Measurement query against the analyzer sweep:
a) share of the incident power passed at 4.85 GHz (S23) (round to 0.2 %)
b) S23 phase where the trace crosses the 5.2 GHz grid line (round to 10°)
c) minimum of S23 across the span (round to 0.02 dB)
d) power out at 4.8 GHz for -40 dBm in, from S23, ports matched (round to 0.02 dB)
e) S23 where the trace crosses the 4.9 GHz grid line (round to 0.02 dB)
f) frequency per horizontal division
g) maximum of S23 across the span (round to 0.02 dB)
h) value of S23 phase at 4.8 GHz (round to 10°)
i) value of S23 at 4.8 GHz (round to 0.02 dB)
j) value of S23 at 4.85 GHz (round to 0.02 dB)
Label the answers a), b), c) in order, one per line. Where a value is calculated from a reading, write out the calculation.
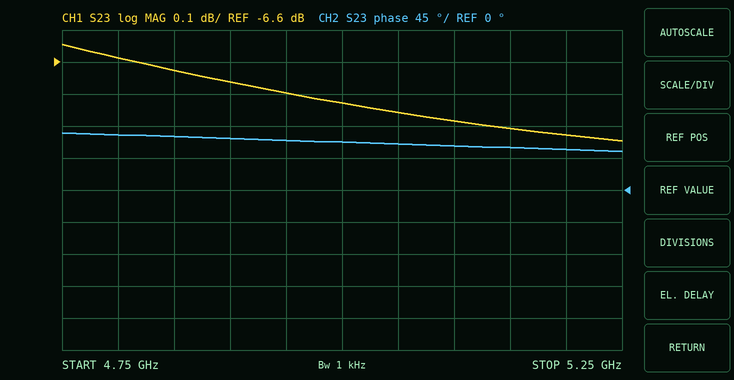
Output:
a) 10^(-6.62/10) ≈ 21.8 %
b) 60°
c) -6.84 dB
d) -40 dBm + (-6.58 dB) = -46.58 dBm
e) -6.66 dB
f) 50 MHz
g) -6.54 dB
h) 80°
i) -6.58 dB
j) -6.62 dB
